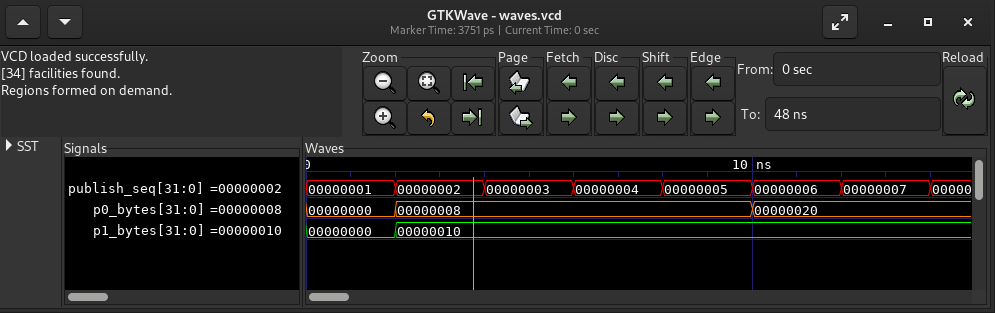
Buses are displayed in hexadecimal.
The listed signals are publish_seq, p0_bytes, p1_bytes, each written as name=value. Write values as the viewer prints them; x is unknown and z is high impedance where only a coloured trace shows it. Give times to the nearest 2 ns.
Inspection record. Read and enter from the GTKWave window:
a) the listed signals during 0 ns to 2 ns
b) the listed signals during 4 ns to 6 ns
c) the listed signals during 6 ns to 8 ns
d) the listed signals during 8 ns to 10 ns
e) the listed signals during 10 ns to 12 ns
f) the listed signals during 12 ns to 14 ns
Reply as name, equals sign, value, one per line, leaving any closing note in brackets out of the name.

the listed signals during 0 ns to 2 ns = publish_seq=00000001, p0_bytes=00000000, p1_bytes=00000000
the listed signals during 4 ns to 6 ns = publish_seq=00000003, p0_bytes=00000008, p1_bytes=00000010
the listed signals during 6 ns to 8 ns = publish_seq=00000004, p0_bytes=00000008, p1_bytes=00000010
the listed signals during 8 ns to 10 ns = publish_seq=00000005, p0_bytes=00000008, p1_bytes=00000010
the listed signals during 10 ns to 12 ns = publish_seq=00000006, p0_bytes=00000020, p1_bytes=00000010
the listed signals during 12 ns to 14 ns = publish_seq=00000007, p0_bytes=00000020, p1_bytes=00000010
